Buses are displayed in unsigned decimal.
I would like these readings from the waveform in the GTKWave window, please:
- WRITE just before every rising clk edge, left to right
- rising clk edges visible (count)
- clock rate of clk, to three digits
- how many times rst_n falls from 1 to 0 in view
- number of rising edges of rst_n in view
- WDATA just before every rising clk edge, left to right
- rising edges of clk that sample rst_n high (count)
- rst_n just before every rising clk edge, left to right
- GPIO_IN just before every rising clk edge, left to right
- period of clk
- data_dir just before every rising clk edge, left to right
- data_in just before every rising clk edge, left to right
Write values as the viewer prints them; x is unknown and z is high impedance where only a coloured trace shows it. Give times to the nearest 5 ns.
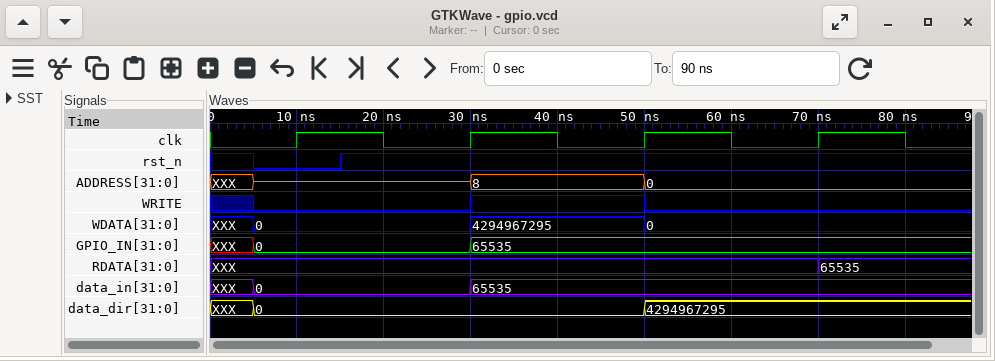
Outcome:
0 0 1 0
4
50.0 MHz
1
1
0, 0, 4294967295, 0
3
0 1 1 1
0, 0, 65535, 65535
20 ns
0, 0, 0, 4294967295
0, 0, 65535, 65535
